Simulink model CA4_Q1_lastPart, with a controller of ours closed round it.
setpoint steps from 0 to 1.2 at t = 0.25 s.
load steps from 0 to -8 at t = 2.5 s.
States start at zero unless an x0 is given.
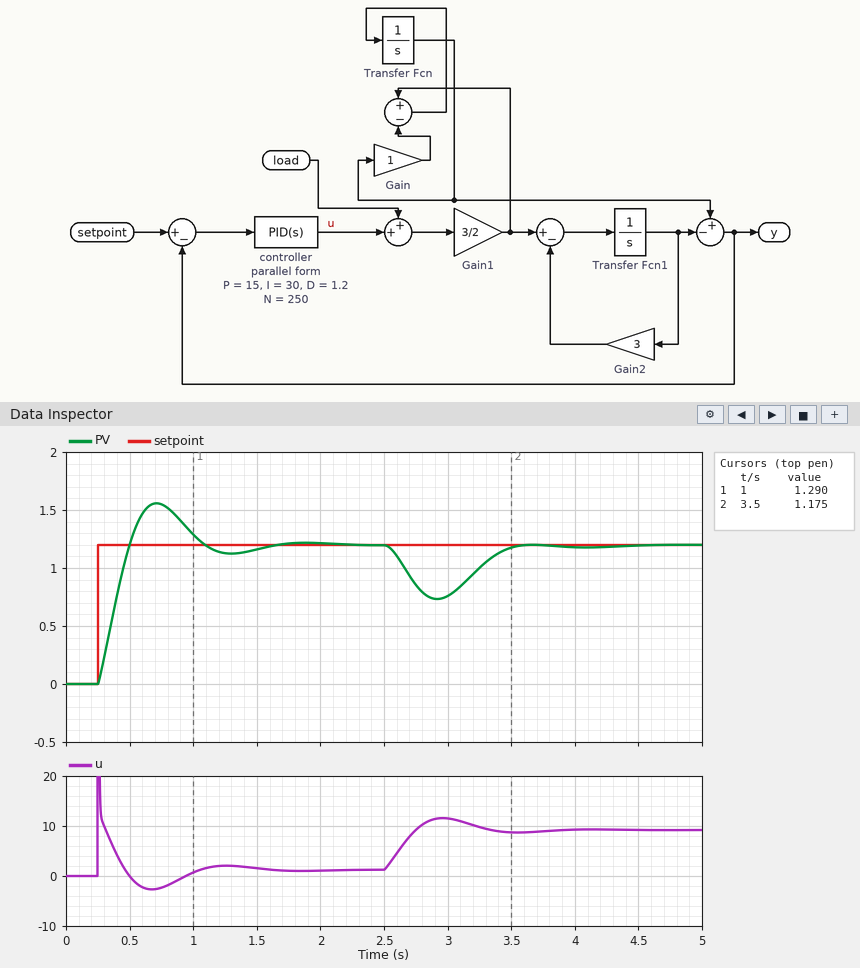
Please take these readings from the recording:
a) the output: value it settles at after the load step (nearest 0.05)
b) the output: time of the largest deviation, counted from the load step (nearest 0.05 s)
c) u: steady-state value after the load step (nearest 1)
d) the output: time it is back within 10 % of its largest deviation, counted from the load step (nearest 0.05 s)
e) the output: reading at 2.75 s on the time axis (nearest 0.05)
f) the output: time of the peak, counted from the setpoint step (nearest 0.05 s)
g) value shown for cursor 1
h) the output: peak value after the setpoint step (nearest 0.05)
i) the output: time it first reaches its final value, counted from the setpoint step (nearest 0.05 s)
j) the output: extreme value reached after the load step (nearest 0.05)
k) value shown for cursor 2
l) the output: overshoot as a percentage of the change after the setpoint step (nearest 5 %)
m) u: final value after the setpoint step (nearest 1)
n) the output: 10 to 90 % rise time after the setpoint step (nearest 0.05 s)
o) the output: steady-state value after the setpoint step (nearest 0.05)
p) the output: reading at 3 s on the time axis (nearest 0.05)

1.20
0.40 s
9
0.95 s
0.85
0.45 s
1.290
1.55
0.25 s
0.75
1.175
30 %
1
0.20 s
1.20
0.75
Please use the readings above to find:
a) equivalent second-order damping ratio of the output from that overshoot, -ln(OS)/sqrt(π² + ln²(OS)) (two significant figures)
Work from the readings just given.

0.36
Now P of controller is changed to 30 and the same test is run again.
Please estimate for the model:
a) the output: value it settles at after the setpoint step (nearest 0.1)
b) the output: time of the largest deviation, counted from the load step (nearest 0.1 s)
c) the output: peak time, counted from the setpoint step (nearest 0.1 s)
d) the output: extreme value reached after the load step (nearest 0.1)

1.2
0.3 s
0.3 s
0.9
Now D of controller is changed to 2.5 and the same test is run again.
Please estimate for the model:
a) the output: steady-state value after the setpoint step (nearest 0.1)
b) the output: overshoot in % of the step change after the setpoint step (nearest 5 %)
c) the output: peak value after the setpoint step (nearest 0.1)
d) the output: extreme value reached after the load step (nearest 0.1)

1.2
15 %
1.4
0.8
